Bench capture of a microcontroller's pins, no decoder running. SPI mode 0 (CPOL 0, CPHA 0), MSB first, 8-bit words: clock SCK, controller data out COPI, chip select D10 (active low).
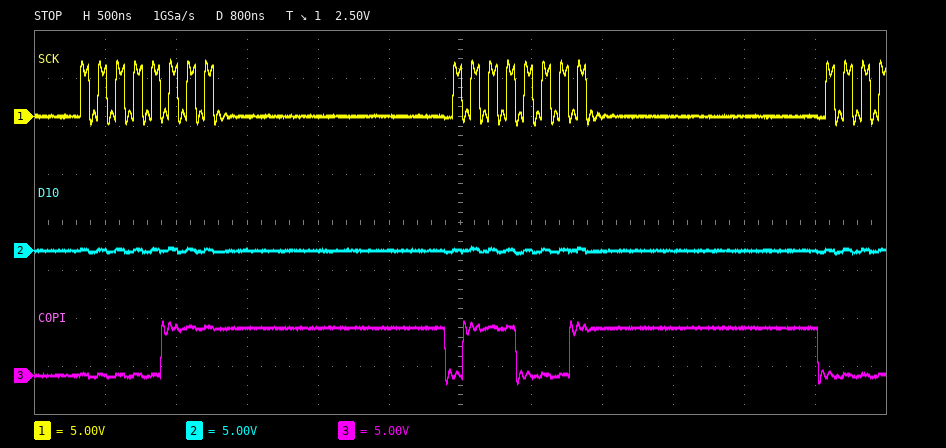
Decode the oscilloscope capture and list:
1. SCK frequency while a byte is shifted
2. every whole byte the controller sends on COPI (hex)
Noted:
8 MHz
0x07 0x71
